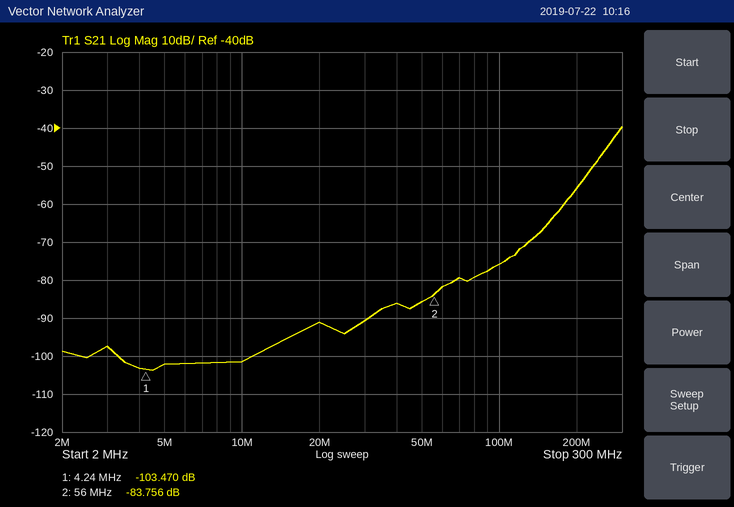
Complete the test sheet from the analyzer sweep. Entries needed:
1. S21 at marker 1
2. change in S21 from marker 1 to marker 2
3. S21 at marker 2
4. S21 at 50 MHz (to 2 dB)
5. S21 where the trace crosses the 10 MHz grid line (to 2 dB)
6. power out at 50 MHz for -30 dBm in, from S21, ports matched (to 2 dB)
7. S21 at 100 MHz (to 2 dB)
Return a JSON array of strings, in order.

["-103.470 dB", "19.714 dB", "-83.756 dB", "-86 dB", "-102 dB", "-116 dBm", "-76 dB"]
